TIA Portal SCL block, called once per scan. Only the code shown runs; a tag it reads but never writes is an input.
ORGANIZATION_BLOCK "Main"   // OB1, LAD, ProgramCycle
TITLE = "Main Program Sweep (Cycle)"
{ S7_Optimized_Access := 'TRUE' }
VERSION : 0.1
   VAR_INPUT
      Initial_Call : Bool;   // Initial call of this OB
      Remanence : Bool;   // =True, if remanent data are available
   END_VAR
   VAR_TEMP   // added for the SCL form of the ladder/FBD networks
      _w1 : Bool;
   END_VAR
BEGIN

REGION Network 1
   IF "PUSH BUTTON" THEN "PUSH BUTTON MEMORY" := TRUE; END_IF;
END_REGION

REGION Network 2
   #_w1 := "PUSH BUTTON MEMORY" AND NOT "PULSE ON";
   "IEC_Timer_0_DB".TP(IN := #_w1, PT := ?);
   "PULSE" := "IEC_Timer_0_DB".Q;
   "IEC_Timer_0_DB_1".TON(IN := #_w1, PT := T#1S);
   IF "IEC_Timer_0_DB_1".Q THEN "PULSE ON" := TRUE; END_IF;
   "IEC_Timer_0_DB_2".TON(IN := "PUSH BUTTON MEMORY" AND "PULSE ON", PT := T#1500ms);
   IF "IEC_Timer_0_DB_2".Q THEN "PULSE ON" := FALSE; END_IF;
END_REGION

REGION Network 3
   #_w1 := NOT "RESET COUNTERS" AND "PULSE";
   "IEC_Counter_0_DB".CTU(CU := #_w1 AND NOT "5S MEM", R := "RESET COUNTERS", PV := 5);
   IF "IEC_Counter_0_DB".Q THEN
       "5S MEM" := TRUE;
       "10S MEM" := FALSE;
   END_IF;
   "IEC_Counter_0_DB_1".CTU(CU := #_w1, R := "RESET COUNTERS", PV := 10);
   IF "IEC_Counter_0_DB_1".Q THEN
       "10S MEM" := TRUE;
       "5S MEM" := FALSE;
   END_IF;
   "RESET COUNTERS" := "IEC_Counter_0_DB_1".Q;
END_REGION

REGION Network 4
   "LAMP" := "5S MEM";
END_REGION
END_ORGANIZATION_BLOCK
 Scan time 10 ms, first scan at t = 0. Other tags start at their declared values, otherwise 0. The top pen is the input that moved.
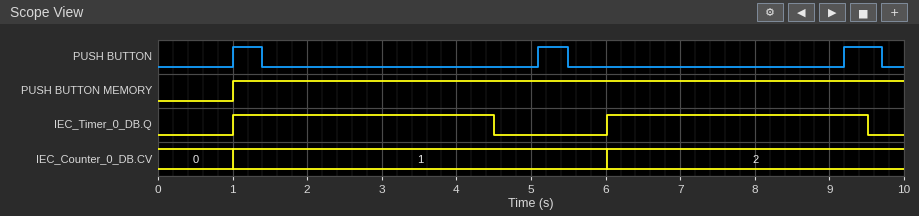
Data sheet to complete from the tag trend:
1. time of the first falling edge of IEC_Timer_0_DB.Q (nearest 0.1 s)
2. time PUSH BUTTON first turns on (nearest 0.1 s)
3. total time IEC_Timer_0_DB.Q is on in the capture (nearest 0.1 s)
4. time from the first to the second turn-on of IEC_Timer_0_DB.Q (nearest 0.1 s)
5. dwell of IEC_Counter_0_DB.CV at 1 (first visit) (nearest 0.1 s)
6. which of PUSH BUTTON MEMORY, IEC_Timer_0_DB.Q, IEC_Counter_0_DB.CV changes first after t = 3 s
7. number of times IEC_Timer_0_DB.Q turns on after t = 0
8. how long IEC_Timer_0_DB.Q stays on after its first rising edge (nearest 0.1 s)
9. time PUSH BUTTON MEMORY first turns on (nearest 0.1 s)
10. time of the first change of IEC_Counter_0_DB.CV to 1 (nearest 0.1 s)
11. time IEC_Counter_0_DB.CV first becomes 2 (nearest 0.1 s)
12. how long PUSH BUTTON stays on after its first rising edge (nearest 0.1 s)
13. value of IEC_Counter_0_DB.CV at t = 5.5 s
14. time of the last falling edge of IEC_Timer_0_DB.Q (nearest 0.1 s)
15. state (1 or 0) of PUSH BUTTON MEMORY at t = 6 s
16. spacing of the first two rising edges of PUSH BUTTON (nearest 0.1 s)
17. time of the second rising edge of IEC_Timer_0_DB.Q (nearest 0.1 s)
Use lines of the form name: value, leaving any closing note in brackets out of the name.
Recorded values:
time of the first falling edge of IEC_Timer_0_DB.Q: 4.5 s
time PUSH BUTTON first turns on: 1.0 s
total time IEC_Timer_0_DB.Q is on in the capture: 7.0 s
time from the first to the second turn-on of IEC_Timer_0_DB.Q: 5.0 s
dwell of IEC_Counter_0_DB.CV at 1 (first visit): 5.0 s
which of PUSH BUTTON MEMORY, IEC_Timer_0_DB.Q, IEC_Counter_0_DB.CV changes first after t = 3 s: IEC_Timer_0_DB.Q
number of times IEC_Timer_0_DB.Q turns on after t = 0: 2
how long IEC_Timer_0_DB.Q stays on after its first rising edge: 3.5 s
time PUSH BUTTON MEMORY first turns on: 1.0 s
time of the first change of IEC_Counter_0_DB.CV to 1: 1.0 s
time IEC_Counter_0_DB.CV first becomes 2: 6.0 s
how long PUSH BUTTON stays on after its first rising edge: 0.4 s
value of IEC_Counter_0_DB.CV at t = 5.5 s: 1
time of the last falling edge of IEC_Timer_0_DB.Q: 9.5 s
state (1 or 0) of PUSH BUTTON MEMORY at t = 6 s: 1
spacing of the first two rising edges of PUSH BUTTON: 4.1 s
time of the second rising edge of IEC_Timer_0_DB.Q: 6.0 s
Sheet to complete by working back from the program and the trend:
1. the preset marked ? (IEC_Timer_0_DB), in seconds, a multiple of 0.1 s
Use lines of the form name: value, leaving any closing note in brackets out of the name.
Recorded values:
the preset marked ? (IEC_Timer_0_DB), in seconds, a multiple of 0.1 s: 3.5 s
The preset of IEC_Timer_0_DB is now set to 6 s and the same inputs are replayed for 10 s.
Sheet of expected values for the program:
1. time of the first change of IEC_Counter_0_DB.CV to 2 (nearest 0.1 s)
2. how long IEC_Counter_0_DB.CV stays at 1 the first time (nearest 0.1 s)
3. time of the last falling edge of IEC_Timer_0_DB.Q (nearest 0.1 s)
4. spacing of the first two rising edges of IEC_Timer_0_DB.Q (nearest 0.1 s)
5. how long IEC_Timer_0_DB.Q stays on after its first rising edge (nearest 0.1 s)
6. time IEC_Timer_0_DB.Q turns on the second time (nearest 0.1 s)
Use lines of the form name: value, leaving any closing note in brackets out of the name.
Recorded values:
time of the first change of IEC_Counter_0_DB.CV to 2: 8.5 s
how long IEC_Counter_0_DB.CV stays at 1 the first time: 7.5 s
time of the last falling edge of IEC_Timer_0_DB.Q: 7.0 s
spacing of the first two rising edges of IEC_Timer_0_DB.Q: 7.5 s
how long IEC_Timer_0_DB.Q stays on after its first rising edge: 6.0 s
time IEC_Timer_0_DB.Q turns on the second time: 8.5 s
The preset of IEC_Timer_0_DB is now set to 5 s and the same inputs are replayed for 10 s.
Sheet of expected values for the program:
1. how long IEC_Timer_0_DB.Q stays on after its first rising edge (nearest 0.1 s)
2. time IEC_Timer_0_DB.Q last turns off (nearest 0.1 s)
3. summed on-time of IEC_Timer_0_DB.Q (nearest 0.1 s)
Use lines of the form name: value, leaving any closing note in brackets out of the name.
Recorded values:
how long IEC_Timer_0_DB.Q stays on after its first rising edge: 5.0 s
time IEC_Timer_0_DB.Q last turns off: 6.0 s
summed on-time of IEC_Timer_0_DB.Q: 9.0 s
